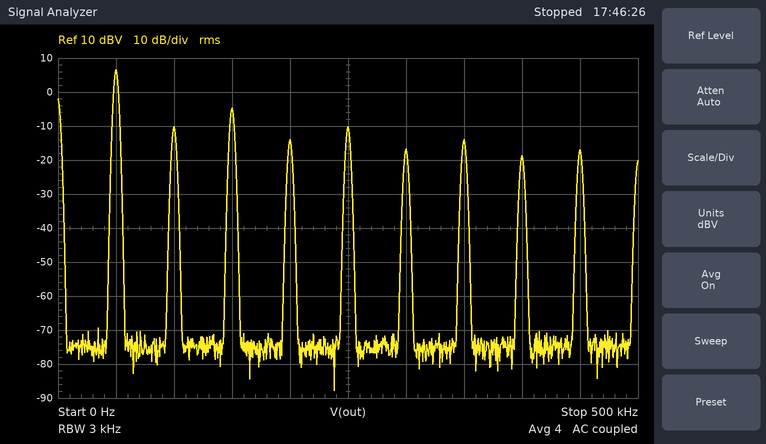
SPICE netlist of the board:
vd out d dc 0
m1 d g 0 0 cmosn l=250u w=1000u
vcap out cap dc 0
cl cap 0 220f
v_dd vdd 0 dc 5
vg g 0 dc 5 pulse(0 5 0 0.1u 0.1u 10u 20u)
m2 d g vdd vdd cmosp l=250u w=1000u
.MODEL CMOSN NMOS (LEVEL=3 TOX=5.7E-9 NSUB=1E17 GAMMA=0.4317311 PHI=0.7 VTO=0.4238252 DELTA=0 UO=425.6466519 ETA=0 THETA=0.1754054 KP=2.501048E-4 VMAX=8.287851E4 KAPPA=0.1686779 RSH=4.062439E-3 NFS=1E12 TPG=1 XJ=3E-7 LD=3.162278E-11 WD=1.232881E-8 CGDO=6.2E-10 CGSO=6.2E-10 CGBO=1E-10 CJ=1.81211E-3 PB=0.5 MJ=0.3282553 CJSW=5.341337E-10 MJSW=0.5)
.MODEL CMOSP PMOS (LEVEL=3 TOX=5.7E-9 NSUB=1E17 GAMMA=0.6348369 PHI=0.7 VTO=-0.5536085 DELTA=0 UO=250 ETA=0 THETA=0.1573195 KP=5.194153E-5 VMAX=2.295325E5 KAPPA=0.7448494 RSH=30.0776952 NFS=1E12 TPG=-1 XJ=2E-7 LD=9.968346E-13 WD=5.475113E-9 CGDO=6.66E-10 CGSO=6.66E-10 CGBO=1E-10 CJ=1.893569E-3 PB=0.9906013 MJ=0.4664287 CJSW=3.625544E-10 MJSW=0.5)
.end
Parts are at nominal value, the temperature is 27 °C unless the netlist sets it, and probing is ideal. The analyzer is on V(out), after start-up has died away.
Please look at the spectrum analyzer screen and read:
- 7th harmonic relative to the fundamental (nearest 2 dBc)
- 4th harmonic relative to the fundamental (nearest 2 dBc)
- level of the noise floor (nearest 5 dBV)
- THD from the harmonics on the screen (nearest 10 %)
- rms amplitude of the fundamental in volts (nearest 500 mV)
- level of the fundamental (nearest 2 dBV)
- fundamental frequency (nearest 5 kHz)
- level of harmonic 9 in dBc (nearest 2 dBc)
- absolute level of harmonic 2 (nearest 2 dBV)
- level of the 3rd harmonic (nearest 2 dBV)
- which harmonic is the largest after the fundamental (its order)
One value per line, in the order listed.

-20 dBc
-20 dBc
-75 dBV
40 %
2.0 V
6 dBV
50 kHz
-24 dBc
-10 dBV
-4 dBV
3
